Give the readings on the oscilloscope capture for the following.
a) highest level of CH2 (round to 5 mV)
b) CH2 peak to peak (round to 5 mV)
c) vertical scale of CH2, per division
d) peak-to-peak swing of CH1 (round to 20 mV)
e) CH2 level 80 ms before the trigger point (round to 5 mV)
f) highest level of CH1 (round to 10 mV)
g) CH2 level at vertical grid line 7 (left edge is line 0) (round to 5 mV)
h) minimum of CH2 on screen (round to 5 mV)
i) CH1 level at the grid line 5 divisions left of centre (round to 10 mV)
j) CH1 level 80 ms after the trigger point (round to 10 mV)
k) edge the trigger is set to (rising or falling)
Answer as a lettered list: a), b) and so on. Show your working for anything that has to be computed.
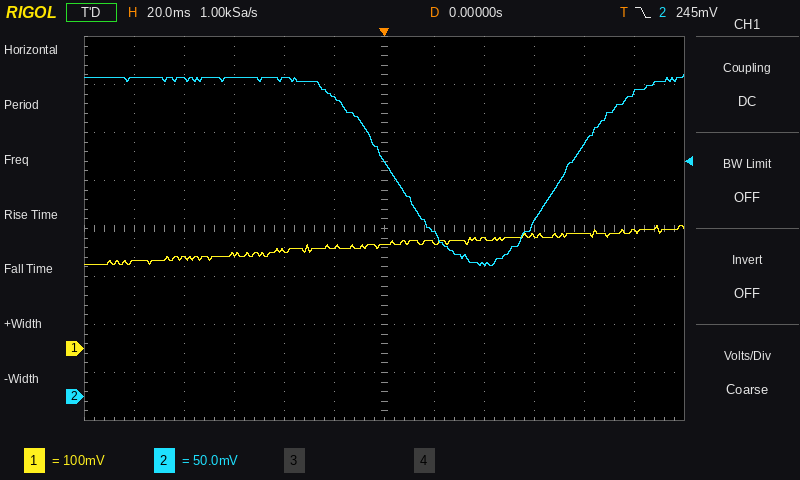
a) 335 mV
b) 335 mV − (135 mV) = 200 mV
c) 50 mV
d) 80 mV
e) 330 mV
f) 260 mV
g) 170 mV
h) 135 mV
i) 180 mV
j) 240 mV
k) falling
